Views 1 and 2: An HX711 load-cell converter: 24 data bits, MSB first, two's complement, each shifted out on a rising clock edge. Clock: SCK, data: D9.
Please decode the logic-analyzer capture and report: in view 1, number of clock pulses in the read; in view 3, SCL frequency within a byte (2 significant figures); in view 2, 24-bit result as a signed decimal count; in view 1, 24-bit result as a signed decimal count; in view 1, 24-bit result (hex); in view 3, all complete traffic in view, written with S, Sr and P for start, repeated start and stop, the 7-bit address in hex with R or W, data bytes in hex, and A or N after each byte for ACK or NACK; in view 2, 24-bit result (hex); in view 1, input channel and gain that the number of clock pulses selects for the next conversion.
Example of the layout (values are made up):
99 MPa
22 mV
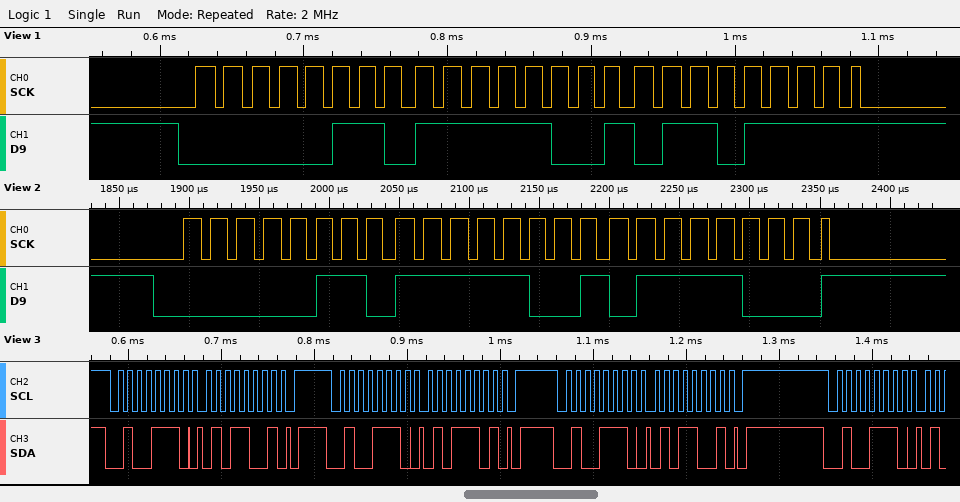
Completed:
25
100 kHz
457080
457071
0x06F96F
S 27W A 59 A P S 27W A 5D A P S 27W A 59 A P S 27W A
0x06F978
channel A, gain 128
